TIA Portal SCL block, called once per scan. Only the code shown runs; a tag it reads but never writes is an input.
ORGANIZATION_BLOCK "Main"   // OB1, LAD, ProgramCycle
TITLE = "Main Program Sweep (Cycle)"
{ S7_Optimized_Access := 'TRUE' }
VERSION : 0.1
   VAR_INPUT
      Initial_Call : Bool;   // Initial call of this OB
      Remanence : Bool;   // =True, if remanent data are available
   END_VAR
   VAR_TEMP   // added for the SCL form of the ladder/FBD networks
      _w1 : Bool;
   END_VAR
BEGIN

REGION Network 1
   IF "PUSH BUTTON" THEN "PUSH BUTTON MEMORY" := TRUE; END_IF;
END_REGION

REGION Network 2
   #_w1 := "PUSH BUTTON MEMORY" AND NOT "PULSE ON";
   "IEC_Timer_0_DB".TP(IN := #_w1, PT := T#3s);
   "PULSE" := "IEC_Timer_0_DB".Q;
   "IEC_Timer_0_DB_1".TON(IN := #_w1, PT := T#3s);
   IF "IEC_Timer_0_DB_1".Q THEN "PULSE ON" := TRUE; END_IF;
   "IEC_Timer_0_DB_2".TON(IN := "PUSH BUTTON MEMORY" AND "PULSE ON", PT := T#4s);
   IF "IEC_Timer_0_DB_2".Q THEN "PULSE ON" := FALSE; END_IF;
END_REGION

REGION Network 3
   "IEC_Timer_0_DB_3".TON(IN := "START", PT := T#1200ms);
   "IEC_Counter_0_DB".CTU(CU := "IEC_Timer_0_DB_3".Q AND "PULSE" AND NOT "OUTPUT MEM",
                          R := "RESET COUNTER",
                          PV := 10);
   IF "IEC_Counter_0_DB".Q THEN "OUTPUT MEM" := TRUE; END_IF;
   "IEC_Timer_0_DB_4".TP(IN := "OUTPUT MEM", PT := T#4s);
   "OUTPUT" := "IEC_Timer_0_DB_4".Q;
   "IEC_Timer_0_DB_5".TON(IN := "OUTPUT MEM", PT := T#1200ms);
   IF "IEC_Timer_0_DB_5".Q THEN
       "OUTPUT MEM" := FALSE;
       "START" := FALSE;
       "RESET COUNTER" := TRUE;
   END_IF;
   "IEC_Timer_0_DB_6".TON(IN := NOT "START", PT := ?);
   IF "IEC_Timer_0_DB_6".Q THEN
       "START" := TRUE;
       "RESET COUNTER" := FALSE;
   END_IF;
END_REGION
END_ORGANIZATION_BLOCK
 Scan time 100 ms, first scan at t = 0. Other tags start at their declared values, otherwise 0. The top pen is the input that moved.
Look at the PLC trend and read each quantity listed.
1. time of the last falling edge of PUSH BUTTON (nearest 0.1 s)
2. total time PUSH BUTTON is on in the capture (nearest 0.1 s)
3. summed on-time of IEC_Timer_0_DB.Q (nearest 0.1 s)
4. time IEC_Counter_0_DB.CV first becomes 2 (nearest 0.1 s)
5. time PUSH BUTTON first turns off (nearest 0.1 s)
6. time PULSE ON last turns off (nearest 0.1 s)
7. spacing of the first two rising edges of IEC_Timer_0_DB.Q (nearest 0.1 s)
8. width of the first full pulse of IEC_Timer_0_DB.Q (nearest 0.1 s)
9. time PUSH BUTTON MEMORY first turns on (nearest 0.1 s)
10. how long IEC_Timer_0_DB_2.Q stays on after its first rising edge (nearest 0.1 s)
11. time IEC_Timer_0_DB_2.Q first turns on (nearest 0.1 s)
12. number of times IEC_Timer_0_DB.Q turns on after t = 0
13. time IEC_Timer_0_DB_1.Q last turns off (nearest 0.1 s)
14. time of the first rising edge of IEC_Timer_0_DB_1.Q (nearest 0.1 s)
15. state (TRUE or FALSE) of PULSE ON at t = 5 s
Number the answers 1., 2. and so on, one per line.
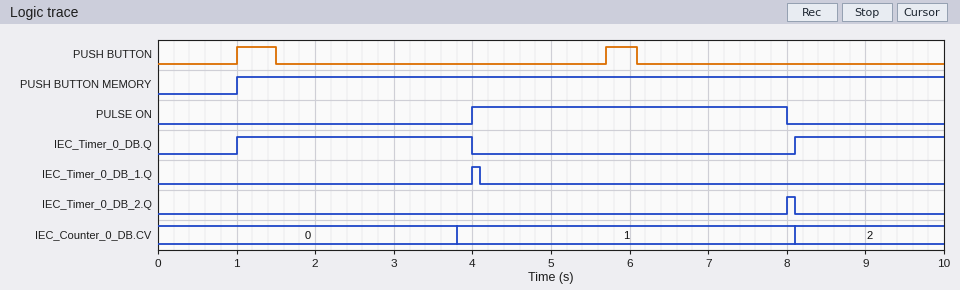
1. 6.1 s
2. 0.9 s
3. 4.9 s
4. 8.1 s
5. 1.5 s
6. 8.0 s
7. 7.1 s
8. 3.0 s
9. 1.0 s
10. 0.1 s
11. 8.0 s
12. 2
13. 4.1 s
14. 4.0 s
15. TRUE
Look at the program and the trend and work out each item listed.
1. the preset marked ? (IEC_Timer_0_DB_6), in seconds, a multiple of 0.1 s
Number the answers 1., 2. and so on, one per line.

1. 2.5 s
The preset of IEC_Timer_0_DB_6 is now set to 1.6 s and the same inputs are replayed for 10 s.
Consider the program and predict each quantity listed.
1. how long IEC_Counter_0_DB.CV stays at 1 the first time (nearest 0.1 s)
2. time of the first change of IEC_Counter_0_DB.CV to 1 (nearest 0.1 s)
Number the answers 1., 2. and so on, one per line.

1. 5.2 s
2. 2.9 s
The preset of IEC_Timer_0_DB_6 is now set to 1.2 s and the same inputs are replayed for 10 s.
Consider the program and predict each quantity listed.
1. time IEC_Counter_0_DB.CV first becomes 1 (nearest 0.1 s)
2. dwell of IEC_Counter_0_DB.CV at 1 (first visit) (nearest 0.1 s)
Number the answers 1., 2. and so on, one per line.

1. 2.5 s
2. 5.6 s
